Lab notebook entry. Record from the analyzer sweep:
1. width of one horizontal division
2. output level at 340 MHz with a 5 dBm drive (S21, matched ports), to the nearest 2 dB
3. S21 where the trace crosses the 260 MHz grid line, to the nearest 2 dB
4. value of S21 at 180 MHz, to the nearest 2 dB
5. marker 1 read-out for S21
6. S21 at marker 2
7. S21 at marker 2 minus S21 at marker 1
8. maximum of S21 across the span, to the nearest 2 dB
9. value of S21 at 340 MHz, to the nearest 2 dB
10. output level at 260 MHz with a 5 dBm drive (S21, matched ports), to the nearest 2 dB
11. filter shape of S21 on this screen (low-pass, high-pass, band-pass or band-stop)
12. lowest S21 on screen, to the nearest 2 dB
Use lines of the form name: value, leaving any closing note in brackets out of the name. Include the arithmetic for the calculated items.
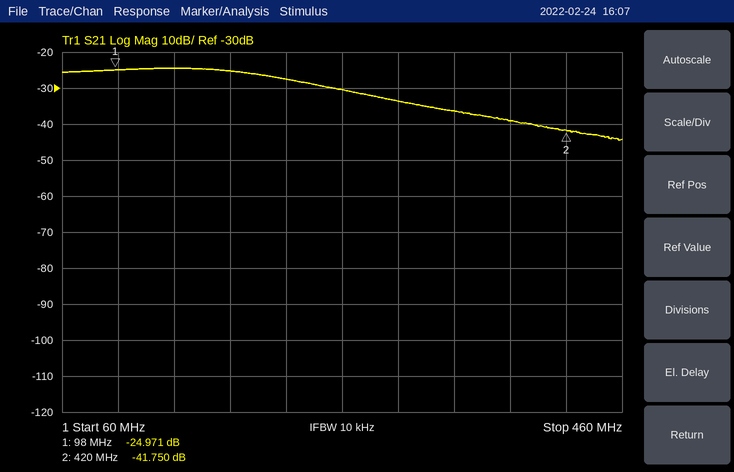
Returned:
width of one horizontal division: 40 MHz
output level at 340 MHz with a 5 dBm drive (S21, matched ports), to the nearest 2 dB: 5 dBm + (-36 dB) = -32 dBm
S21 where the trace crosses the 260 MHz grid line, to the nearest 2 dB: -30 dB
value of S21 at 180 MHz, to the nearest 2 dB: -26 dB
marker 1 read-out for S21: -24.971 dB
S21 at marker 2: -41.750 dB
S21 at marker 2 minus S21 at marker 1: -41.75 − (-24.971) = -16.779 dB
maximum of S21 across the span, to the nearest 2 dB: -24 dB
value of S21 at 340 MHz, to the nearest 2 dB: -36 dB
output level at 260 MHz with a 5 dBm drive (S21, matched ports), to the nearest 2 dB: 5 dBm + (-30 dB) = -26 dBm
filter shape of S21 on this screen: low-pass
lowest S21 on screen, to the nearest 2 dB: -44 dB
